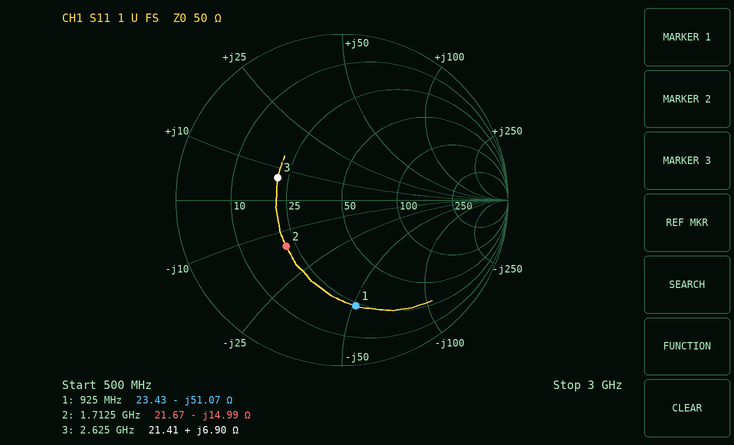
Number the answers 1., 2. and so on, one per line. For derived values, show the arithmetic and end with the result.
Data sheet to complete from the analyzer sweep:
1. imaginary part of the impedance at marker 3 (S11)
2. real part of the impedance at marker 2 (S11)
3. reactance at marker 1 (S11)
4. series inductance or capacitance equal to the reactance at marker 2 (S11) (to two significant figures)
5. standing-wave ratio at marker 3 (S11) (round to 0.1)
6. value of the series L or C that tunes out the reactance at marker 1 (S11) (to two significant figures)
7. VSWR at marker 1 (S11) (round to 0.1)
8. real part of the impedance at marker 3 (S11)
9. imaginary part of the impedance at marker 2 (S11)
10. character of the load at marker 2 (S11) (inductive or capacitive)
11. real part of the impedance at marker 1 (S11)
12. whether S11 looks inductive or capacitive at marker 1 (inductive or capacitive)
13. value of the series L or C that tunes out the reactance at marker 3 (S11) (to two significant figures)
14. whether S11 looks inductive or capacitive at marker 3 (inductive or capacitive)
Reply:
1. +6.90 Ω
2. 21.67 Ω
3. -51.07 Ω
4. C = 1/(2π × 1.7125 GHz × 14.99 Ω) ≈ 6.2 pF
5. 2.4
6. L = 51.07 Ω/(2π × 925 MHz) ≈ 8.8 nH
7. 4.6
8. 21.41 Ω
9. -14.99 Ω
10. capacitive
11. 23.43 Ω
12. capacitive
13. C = 1/(2π × 2.625 GHz × 6.9 Ω) ≈ 8.8 pF
14. inductive
